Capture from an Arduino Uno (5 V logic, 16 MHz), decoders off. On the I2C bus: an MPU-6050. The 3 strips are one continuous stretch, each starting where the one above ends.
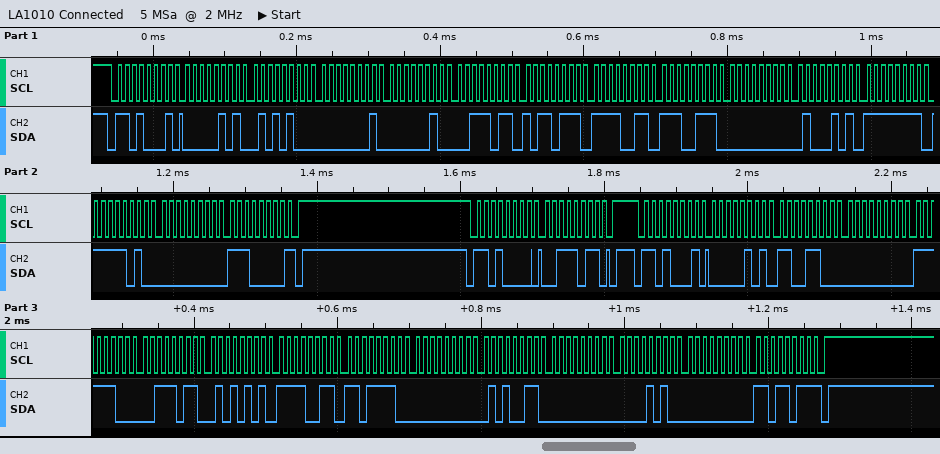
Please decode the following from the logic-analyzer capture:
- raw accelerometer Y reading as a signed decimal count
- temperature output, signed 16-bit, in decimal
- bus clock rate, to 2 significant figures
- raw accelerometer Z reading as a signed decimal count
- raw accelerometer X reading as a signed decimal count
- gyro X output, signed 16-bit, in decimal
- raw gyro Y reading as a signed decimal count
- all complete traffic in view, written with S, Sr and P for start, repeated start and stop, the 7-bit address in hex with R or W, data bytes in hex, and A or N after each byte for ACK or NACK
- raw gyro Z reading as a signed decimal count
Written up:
252
-3106
100 kHz
15189
1484
83
10
S 68R A 05 A 54 A 01 A 02 A 3B A B7 A F3 A E7 A 00 A 45 A FF A FA A 00 A E0 N P S 68W A 3B A P S 68R A 05 A CC A 00 A FC A 3B A 55 A F3 A DE A 00 A 53 A 00 A 0A A 00 A DB N P
219
